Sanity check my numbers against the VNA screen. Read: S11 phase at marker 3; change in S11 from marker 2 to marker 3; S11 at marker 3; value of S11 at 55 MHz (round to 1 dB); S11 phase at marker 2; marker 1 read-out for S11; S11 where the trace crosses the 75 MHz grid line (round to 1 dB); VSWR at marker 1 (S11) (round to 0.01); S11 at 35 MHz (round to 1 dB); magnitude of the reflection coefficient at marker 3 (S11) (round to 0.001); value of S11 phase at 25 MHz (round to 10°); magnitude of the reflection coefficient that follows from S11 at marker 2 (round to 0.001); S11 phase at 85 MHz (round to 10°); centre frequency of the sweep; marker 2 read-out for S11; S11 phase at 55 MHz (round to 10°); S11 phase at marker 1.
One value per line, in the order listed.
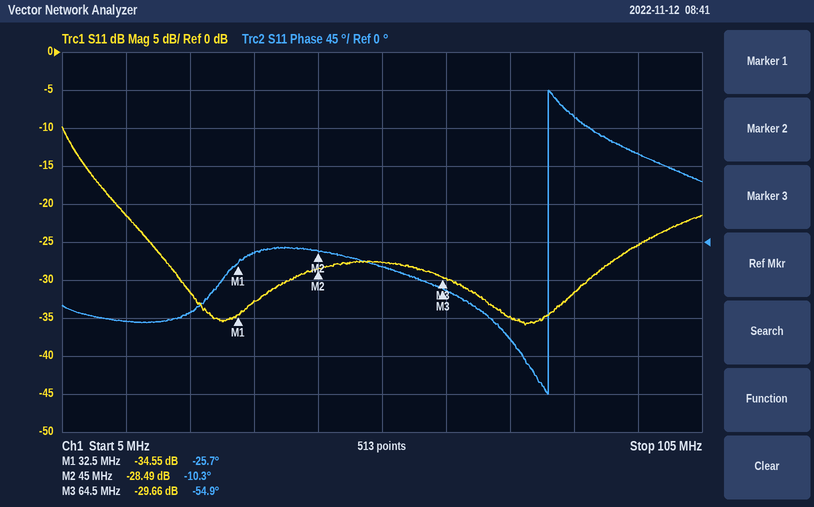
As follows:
-54.9°
-1.17 dB
-29.66 dB
-28 dB
-10.3°
-34.55 dB
-35 dB
1.04
-33 dB
0.033
-80°
0.038
150°
55 MHz
-28.49 dB
-30°
-25.7°
